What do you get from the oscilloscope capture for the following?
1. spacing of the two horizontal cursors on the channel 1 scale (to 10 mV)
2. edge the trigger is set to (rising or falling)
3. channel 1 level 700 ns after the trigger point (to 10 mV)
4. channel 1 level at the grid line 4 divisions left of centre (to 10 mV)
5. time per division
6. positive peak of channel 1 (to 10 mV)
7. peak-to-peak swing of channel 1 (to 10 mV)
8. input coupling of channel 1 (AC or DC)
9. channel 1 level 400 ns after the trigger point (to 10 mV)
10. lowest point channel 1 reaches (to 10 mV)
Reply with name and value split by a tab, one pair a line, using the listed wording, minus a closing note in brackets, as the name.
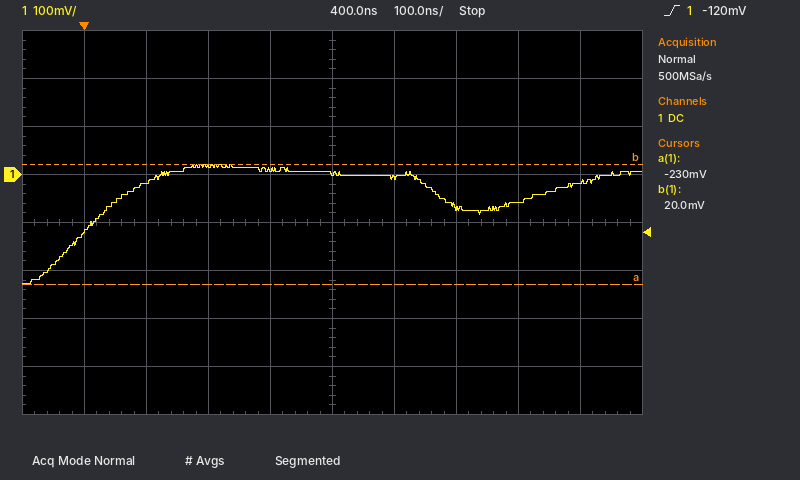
spacing of the two horizontal cursors on the channel 1 scale	250 mV
edge the trigger is set to	rising
channel 1 level 700 ns after the trigger point	-60 mV
channel 1 level at the grid line 4 divisions left of centre	-120 mV
time per division	100 ns
positive peak of channel 1	20 mV
peak-to-peak swing of channel 1	250 mV
input coupling of channel 1	DC
channel 1 level 400 ns after the trigger point	0 mV
lowest point channel 1 reaches	-230 mV
